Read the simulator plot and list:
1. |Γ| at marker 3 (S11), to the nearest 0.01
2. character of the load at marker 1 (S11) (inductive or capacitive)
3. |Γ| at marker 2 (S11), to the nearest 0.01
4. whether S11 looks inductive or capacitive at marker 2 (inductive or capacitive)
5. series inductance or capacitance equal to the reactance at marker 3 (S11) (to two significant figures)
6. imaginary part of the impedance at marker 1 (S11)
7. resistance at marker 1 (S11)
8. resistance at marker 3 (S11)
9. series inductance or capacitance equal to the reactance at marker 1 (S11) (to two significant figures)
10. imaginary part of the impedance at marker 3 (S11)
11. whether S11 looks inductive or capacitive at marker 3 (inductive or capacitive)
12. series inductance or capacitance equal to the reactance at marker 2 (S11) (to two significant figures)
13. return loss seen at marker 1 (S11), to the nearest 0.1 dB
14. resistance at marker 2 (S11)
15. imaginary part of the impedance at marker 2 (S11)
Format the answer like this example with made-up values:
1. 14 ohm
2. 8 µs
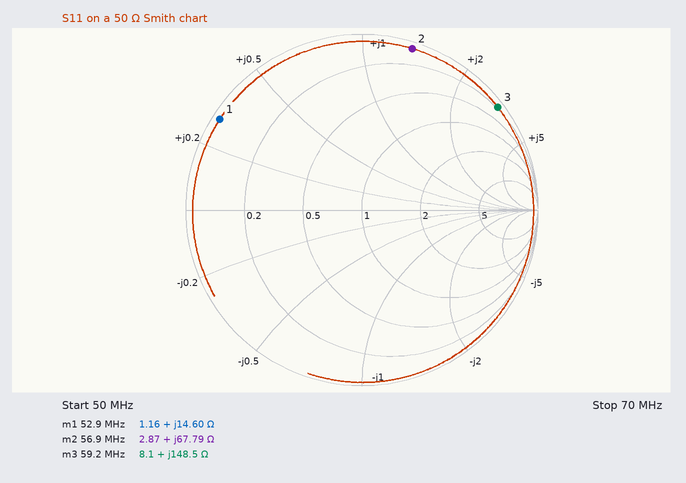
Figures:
1. 0.97
2. inductive
3. 0.96
4. inductive
5. 400 nH
6. +14.60 Ω
7. 1.16 Ω
8. 8.1 Ω
9. 44 nH
10. +148.5 Ω
11. inductive
12. 190 nH
13. 0.4 dB
14. 2.87 Ω
15. +67.79 Ω
